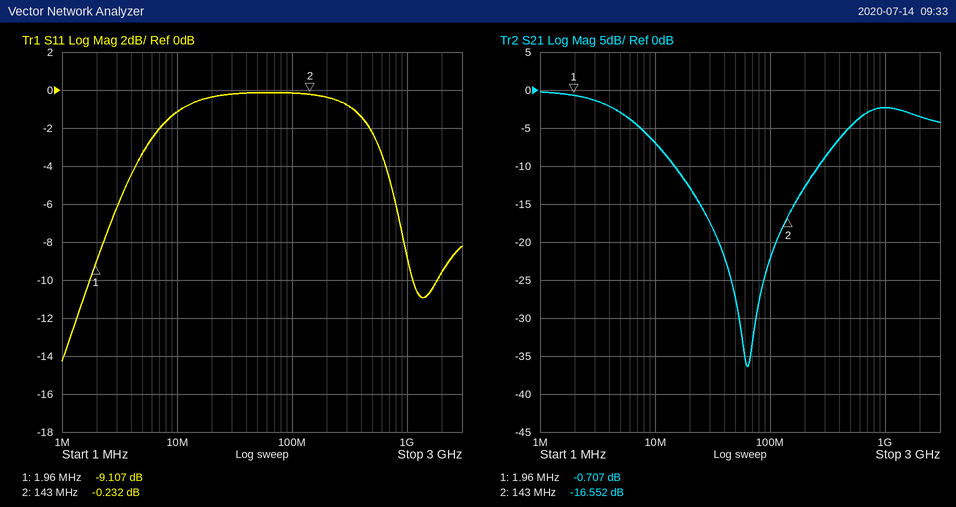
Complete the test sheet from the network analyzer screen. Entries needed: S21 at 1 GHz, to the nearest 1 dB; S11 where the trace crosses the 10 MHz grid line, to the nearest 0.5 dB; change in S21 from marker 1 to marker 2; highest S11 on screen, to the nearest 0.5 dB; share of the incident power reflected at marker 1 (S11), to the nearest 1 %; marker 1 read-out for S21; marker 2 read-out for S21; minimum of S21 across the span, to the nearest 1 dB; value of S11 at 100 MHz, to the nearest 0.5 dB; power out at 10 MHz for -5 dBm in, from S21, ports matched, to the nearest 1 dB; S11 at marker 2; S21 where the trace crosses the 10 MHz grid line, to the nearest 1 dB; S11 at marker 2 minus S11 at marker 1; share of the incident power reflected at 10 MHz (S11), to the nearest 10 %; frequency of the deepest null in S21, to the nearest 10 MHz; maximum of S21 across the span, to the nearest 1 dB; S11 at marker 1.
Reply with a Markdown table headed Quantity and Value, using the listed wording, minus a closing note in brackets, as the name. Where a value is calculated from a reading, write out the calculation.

| Quantity | Value |
|---|---|
| S21 at 1 GHz, to the nearest 1 dB | -2 dB |
| S11 where the trace crosses the 10 MHz grid line, to the nearest 0.5 dB | -1.0 dB |
| change in S21 from marker 1 to marker 2 | -16.552 − (-0.707) = -15.845 dB |
| highest S11 on screen, to the nearest 0.5 dB | 0.0 dB |
| share of the incident power reflected at marker 1 (S11), to the nearest 1 % | 10^(-9.107/10) ≈ 12 % |
| marker 1 read-out for S21 | -0.707 dB |
| marker 2 read-out for S21 | -16.552 dB |
| minimum of S21 across the span, to the nearest 1 dB | -36 dB |
| value of S11 at 100 MHz, to the nearest 0.5 dB | 0.0 dB |
| power out at 10 MHz for -5 dBm in, from S21, ports matched, to the nearest 1 dB | -5 dBm + (-7 dB) = -12 dBm |
| S11 at marker 2 | -0.232 dB |
| S21 where the trace crosses the 10 MHz grid line, to the nearest 1 dB | -7 dB |
| S11 at marker 2 minus S11 at marker 1 | -0.232 − (-9.107) = 8.875 dB |
| share of the incident power reflected at 10 MHz (S11), to the nearest 10 % | 10^(-1/10) ≈ 79.4 %, so 80 % to the nearest 10 % |
| frequency of the deepest null in S21, to the nearest 10 MHz | 60 MHz |
| maximum of S21 across the span, to the nearest 1 dB | 0 dB |
| S11 at marker 1 | -9.107 dB |
